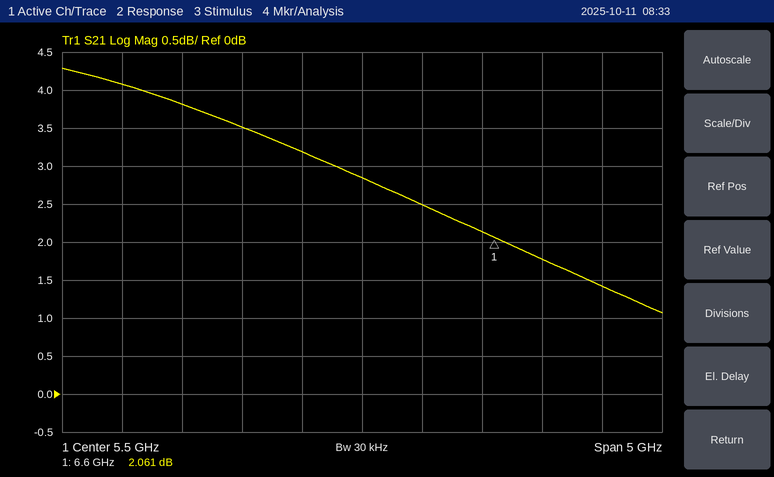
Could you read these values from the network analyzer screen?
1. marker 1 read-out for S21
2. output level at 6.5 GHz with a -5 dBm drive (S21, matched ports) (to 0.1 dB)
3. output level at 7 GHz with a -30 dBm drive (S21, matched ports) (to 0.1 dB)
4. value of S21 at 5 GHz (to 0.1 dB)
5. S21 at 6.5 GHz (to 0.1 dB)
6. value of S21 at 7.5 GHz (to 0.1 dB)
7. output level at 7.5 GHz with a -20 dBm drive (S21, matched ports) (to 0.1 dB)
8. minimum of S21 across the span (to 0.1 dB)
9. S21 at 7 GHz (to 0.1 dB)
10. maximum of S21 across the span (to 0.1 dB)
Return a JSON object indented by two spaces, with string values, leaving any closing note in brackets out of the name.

{
  "marker 1 read-out for S21": "2.061 dB",
  "output level at 6.5 GHz with a -5 dBm drive (S21, matched ports)": "-2.9 dBm",
  "output level at 7 GHz with a -30 dBm drive (S21, matched ports)": "-28.2 dBm",
  "value of S21 at 5 GHz": "3.2 dB",
  "S21 at 6.5 GHz": "2.1 dB",
  "value of S21 at 7.5 GHz": "1.4 dB",
  "output level at 7.5 GHz with a -20 dBm drive (S21, matched ports)": "-18.6 dBm",
  "minimum of S21 across the span": "1.1 dB",
  "S21 at 7 GHz": "1.8 dB",
  "maximum of S21 across the span": "4.3 dB"
}
